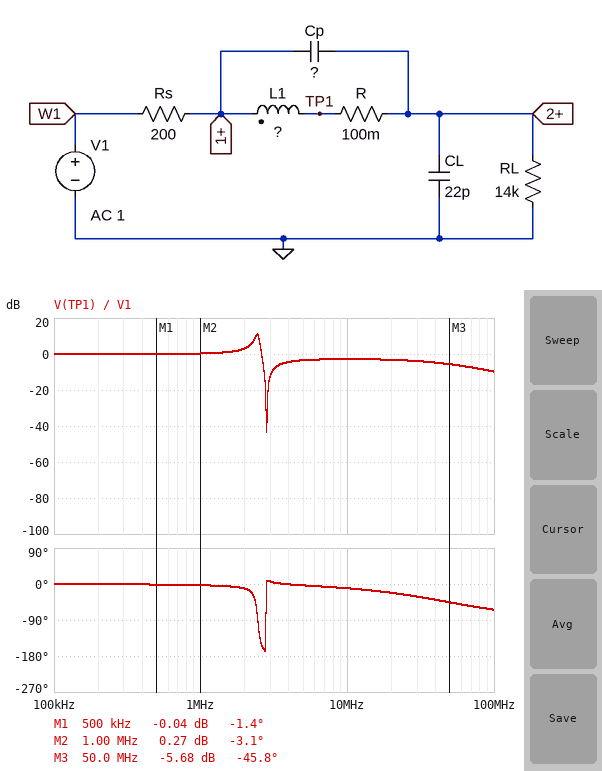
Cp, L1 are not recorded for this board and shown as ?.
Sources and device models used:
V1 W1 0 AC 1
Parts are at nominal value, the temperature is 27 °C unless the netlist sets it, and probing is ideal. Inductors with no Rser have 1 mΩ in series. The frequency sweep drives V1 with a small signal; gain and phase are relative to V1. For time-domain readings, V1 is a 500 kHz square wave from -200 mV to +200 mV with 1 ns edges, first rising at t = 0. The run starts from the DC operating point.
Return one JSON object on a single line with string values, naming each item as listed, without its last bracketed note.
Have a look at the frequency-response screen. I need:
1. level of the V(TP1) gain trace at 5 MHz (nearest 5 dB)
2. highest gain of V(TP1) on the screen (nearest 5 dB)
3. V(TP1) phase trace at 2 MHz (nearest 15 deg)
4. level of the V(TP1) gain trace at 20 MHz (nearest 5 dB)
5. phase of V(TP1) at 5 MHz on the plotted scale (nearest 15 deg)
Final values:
{"level of the V(TP1) gain trace at 5 MHz": "-5 dB", "highest gain of V(TP1) on the screen": "10 dB", "V(TP1) phase trace at 2 MHz": "-15 deg", "level of the V(TP1) gain trace at 20 MHz": "-5 dB", "phase of V(TP1) at 5 MHz on the plotted scale": "0 deg"}
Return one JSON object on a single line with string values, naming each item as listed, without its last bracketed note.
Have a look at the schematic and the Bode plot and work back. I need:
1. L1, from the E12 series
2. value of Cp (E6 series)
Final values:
{"L1, from the E12 series": "47 µH", "value of Cp": "68 pF"}
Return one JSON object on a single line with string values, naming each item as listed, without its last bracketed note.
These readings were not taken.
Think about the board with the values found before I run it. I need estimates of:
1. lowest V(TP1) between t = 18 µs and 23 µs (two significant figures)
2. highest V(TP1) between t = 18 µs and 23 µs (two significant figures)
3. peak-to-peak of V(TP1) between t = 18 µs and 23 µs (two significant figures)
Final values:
{"lowest V(TP1) between t = 18 µs and 23 µs": "-380 mV", "highest V(TP1) between t = 18 µs and 23 µs": "380 mV", "peak-to-peak of V(TP1) between t = 18 µs and 23 µs": "760 mV"}
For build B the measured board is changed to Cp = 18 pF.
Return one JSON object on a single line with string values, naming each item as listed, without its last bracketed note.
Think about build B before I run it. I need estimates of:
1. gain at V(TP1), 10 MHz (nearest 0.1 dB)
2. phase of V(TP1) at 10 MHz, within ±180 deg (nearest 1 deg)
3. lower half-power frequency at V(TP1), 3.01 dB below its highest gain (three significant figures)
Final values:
{"gain at V(TP1), 10 MHz": "-8.8 dB", "phase of V(TP1) at 10 MHz, within ±180 deg": "-4 deg", "lower half-power frequency at V(TP1), 3.01 dB below its highest gain": "3.36 MHz"}
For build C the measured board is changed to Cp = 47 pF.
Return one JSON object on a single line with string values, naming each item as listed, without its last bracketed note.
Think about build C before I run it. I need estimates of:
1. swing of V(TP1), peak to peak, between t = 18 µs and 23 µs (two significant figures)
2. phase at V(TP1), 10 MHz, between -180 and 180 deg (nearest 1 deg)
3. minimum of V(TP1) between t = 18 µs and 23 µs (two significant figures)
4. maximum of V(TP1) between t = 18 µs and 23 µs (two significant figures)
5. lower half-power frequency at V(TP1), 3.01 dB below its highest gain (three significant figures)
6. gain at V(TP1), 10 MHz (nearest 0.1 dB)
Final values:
{"swing of V(TP1), peak to peak, between t = 18 µs and 23 µs": "570 mV", "phase at V(TP1), 10 MHz, between -180 and 180 deg": "-9 deg", "minimum of V(TP1) between t = 18 µs and 23 µs": "-290 mV", "maximum of V(TP1) between t = 18 µs and 23 µs": "290 mV", "lower half-power frequency at V(TP1), 3.01 dB below its highest gain": "2.63 MHz", "gain at V(TP1), 10 MHz": "-3.9 dB"}
